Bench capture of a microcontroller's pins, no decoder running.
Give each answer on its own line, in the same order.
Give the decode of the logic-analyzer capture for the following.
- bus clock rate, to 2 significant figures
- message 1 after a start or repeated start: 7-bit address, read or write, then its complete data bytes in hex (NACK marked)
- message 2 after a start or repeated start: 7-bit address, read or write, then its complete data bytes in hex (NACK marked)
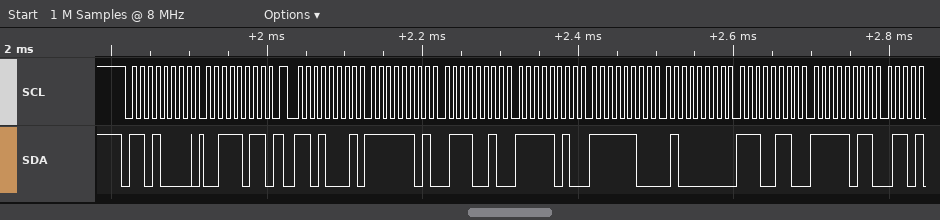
100 kHz
0x68 write: 3B
0x68 read: FD 72 FA FC 40 E6 FB
